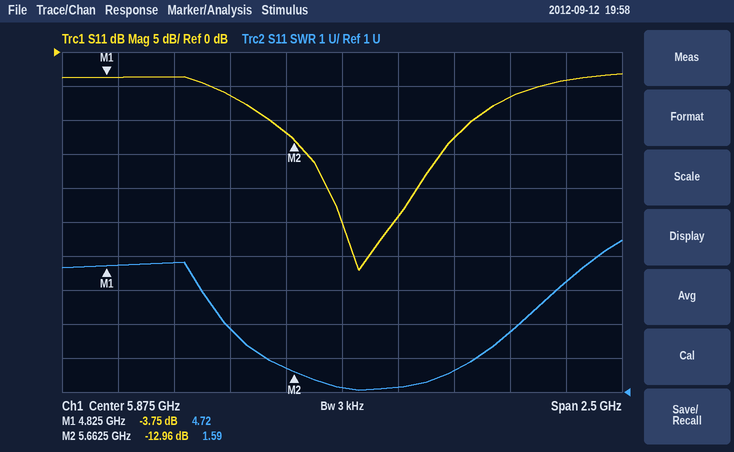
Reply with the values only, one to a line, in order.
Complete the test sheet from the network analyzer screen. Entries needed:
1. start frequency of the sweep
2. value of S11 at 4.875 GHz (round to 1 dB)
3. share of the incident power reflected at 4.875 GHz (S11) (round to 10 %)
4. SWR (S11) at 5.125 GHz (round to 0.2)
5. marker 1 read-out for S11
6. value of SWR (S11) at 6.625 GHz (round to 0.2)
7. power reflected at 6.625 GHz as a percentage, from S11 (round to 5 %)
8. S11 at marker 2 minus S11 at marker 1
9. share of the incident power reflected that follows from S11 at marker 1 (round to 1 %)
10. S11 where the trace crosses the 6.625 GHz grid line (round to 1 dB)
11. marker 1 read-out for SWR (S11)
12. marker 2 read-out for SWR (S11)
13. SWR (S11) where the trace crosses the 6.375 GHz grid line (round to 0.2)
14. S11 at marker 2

4.625 GHz
-4 dB
40 %
4.8
-3.75 dB
2.8
20 %
-9.21 dB
42 %
-7 dB
4.72
1.59
1.6
-12.96 dB
